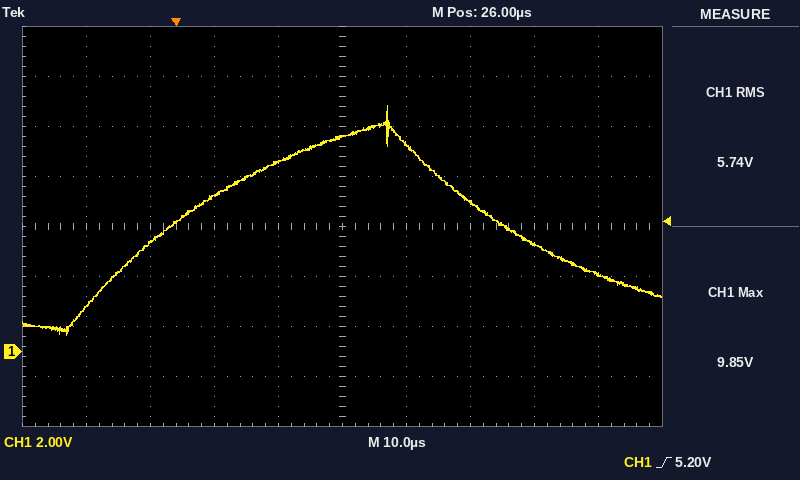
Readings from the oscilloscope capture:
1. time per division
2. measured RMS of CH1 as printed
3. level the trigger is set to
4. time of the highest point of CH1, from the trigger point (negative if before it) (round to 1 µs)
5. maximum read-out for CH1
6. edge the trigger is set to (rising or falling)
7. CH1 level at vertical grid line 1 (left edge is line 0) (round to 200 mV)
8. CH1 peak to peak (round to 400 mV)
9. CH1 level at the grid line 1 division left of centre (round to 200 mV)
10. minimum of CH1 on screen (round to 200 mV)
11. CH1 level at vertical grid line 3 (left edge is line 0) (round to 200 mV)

10 µs
5.74 V
5.20 V
+33 µs
9.85 V
rising
1.8 V
9.2 V
7.6 V
600 mV
6.2 V
